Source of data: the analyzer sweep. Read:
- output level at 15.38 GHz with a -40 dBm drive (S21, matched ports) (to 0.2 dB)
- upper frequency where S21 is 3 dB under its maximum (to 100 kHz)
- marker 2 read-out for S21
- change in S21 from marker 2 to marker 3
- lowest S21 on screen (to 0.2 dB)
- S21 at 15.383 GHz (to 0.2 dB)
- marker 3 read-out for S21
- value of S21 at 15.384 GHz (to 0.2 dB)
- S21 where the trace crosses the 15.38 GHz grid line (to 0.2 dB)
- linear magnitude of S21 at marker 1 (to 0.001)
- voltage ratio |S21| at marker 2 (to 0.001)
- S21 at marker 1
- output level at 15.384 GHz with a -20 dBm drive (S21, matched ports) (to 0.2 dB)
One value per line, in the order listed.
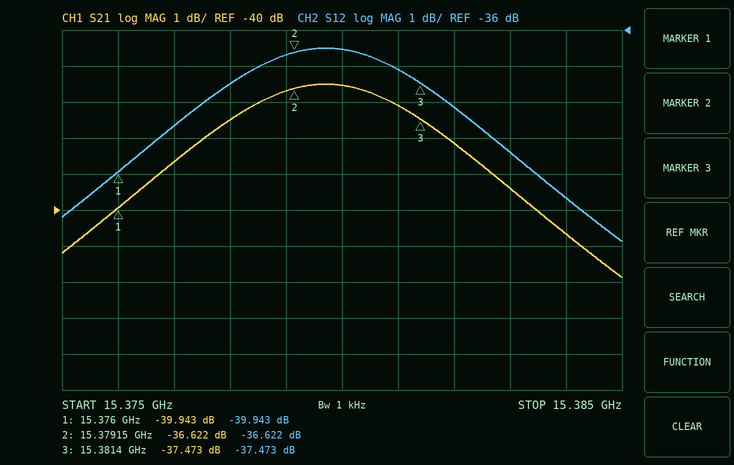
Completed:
-76.6 dBm
15.3831 GHz
-36.622 dB
-0.851 dB
-41.8 dB
-39.4 dB
-37.473 dB
-40.6 dB
-36.6 dB
0.010
0.015
-39.943 dB
-60.6 dBm
